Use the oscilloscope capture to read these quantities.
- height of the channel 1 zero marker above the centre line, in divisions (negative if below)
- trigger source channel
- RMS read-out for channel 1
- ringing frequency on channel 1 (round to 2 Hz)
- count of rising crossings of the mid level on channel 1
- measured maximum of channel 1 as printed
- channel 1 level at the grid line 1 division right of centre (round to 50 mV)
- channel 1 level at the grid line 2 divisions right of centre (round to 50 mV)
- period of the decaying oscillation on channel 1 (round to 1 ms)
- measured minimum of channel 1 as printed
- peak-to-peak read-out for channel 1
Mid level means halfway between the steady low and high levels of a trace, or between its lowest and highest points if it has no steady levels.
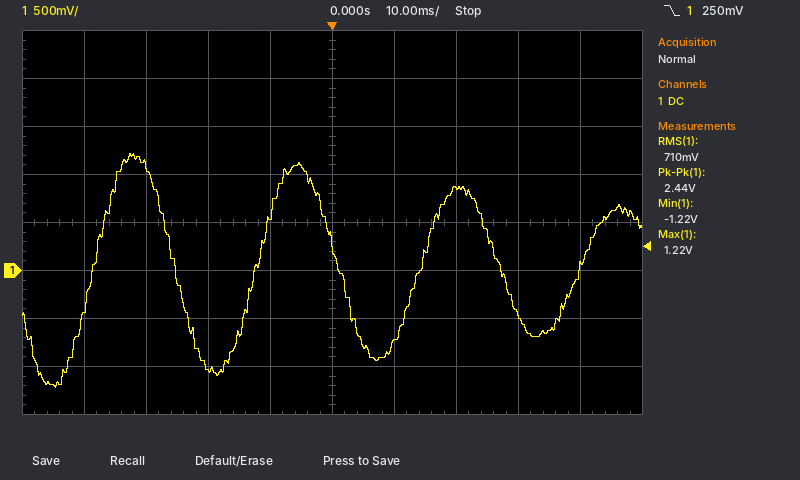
-1.0 div
channel 1
710 mV
38 Hz
4
1.22 V
-750 mV
850 mV
26 ms
-1.22 V
2.44 V
